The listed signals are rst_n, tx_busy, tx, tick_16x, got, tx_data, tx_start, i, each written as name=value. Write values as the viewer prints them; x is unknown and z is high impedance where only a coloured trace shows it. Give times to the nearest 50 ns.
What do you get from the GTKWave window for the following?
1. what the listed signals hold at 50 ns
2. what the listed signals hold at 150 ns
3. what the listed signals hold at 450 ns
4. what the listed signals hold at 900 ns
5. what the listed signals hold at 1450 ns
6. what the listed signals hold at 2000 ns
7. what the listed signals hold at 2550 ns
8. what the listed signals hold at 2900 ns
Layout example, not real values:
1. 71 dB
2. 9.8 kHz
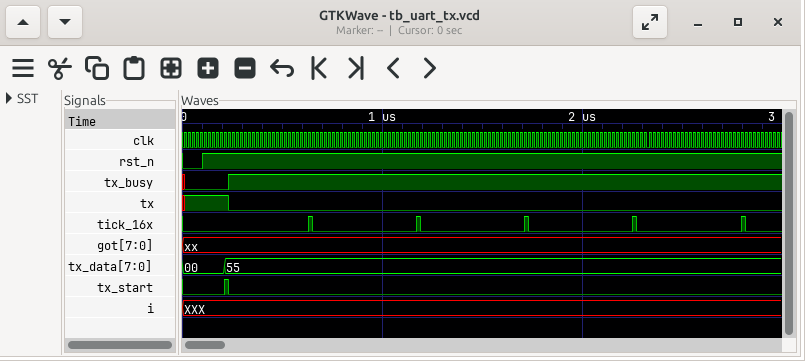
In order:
1. rst_n=0, tx_busy=0, tx=1, tick_16x=0, got=xx, tx_data=00, tx_start=0, i=XXX
2. rst_n=1, tx_busy=0, tx=1, tick_16x=0, got=xx, tx_data=00, tx_start=0, i=XXX
3. rst_n=1, tx_busy=1, tx=0, tick_16x=0, got=xx, tx_data=55, tx_start=0, i=XXX
4. rst_n=1, tx_busy=1, tx=0, tick_16x=0, got=xx, tx_data=55, tx_start=0, i=XXX
5. rst_n=1, tx_busy=1, tx=0, tick_16x=0, got=xx, tx_data=55, tx_start=0, i=XXX
6. rst_n=1, tx_busy=1, tx=0, tick_16x=0, got=xx, tx_data=55, tx_start=0, i=XXX
7. rst_n=1, tx_busy=1, tx=0, tick_16x=0, got=xx, tx_data=55, tx_start=0, i=XXX
8. rst_n=1, tx_busy=1, tx=0, tick_16x=0, got=xx, tx_data=55, tx_start=0, i=XXX
